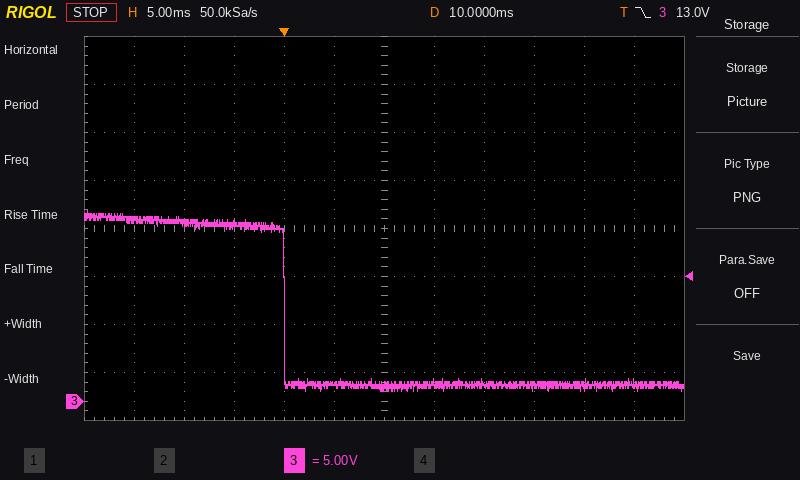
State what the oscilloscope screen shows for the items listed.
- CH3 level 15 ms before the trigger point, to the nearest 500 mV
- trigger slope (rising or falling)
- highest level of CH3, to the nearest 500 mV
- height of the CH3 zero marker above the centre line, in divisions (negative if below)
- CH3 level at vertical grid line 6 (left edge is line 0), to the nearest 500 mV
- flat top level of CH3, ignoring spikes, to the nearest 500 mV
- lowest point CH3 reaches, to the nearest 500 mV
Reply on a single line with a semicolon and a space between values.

19.0 V; falling; 20.0 V; -3.6 div; 1.5 V; 18.5 V; 1.0 V
